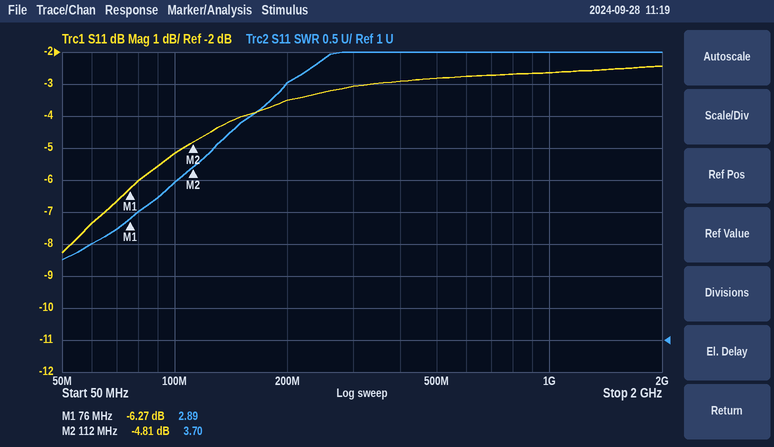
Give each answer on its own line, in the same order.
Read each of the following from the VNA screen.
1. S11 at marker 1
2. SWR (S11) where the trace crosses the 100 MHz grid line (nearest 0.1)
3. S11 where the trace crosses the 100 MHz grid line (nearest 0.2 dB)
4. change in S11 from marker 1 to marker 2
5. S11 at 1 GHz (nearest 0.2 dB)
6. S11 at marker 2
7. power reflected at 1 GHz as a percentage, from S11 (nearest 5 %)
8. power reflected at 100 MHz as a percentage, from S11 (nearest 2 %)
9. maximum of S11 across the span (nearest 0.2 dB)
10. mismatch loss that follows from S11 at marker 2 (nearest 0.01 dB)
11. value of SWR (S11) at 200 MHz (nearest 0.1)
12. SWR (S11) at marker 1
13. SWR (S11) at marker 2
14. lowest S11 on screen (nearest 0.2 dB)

-6.27 dB
3.5
-5.2 dB
1.46 dB
-2.6 dB
-4.81 dB
55 %
30 %
-2.4 dB
1.74 dB
5.0
2.89
3.70
-8.2 dB
